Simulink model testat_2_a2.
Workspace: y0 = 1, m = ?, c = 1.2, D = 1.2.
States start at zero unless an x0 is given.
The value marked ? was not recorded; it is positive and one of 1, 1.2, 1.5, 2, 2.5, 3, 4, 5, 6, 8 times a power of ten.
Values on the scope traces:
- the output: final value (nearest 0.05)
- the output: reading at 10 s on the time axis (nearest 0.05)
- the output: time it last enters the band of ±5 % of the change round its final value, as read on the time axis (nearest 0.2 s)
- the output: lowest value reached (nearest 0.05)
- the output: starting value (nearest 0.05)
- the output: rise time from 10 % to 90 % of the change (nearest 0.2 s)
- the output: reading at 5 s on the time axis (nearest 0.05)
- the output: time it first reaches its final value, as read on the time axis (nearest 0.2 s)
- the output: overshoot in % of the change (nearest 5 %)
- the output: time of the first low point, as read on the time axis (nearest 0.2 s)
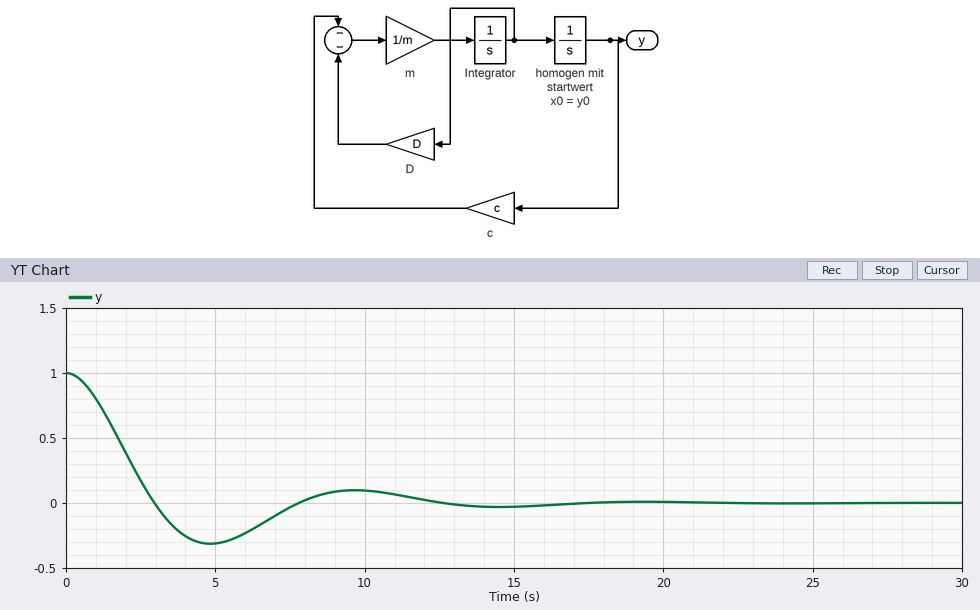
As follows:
0.00
0.10
11.4 s
-0.30
1.00
2.0 s
-0.30
3.0 s
30 %
4.8 s
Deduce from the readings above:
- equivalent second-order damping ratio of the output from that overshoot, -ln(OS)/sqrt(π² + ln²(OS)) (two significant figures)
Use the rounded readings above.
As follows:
0.36
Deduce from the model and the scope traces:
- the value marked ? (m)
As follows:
2.5
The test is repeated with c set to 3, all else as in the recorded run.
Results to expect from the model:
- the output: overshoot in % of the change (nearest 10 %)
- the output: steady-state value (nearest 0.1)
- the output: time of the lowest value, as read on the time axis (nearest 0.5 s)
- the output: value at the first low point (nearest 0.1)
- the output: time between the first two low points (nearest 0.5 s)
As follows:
50 %
0.0
3.0 s
-0.5
6.0 s
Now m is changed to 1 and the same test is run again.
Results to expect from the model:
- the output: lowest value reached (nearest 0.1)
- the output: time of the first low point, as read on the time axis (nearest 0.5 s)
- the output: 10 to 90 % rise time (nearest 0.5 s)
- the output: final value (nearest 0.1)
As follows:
-0.1
3.5 s
1.5 s
0.0
